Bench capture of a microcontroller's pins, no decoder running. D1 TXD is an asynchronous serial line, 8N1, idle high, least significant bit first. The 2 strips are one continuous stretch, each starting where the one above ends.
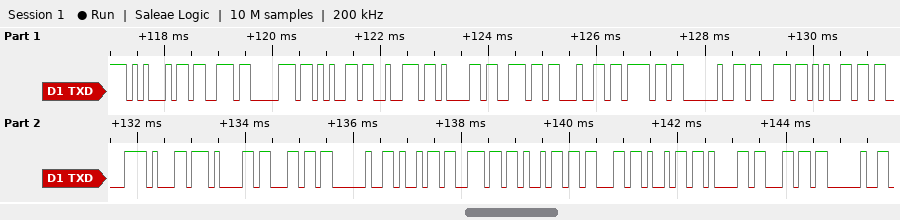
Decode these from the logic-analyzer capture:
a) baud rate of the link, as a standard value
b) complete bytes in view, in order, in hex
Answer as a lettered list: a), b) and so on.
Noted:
a) 9600 baud
b) 0x45 0x73 0x70 0x65 0x72 0x61 0x6E 0x64 0x6F 0x20 0x73 0x65 0xC3 0xB1 0x61 0x6C 0x20 0x69 0x6E 0x69 0x63 0x69 0x61 0x6C 0x20
